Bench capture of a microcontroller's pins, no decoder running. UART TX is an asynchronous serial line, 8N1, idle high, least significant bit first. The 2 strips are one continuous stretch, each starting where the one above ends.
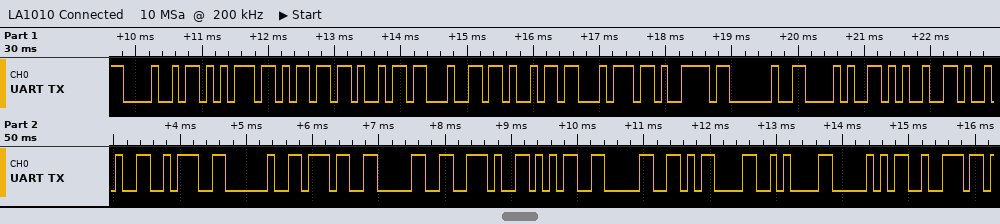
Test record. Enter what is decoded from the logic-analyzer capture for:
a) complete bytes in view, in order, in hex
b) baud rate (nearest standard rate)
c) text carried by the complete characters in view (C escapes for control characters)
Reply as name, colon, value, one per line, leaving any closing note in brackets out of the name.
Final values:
complete bytes in view, in order, in hex: 48 75 6D 69 64 69 74 79 20 28 25 29 3A 20 37 30 2E 35 30 0D 0A 50 72
baud rate: 9600 baud
text carried by the complete characters in view: "Humidity (%): 70.50\r\nPr"
